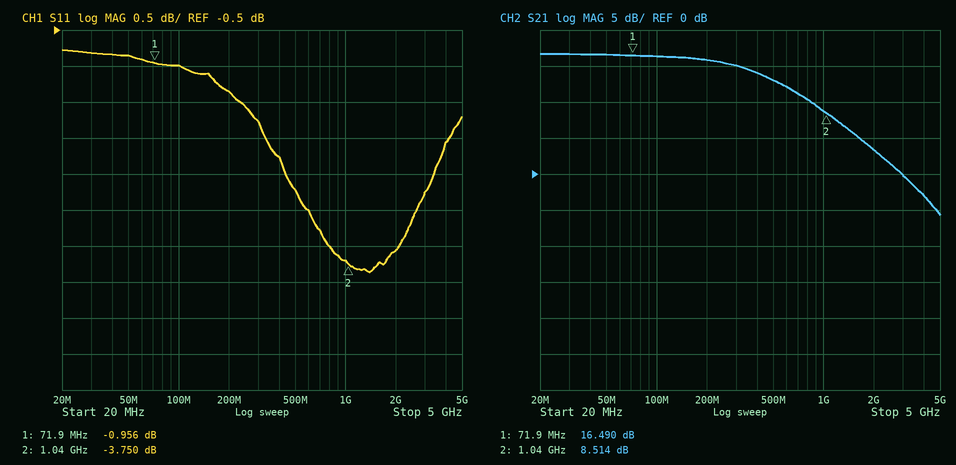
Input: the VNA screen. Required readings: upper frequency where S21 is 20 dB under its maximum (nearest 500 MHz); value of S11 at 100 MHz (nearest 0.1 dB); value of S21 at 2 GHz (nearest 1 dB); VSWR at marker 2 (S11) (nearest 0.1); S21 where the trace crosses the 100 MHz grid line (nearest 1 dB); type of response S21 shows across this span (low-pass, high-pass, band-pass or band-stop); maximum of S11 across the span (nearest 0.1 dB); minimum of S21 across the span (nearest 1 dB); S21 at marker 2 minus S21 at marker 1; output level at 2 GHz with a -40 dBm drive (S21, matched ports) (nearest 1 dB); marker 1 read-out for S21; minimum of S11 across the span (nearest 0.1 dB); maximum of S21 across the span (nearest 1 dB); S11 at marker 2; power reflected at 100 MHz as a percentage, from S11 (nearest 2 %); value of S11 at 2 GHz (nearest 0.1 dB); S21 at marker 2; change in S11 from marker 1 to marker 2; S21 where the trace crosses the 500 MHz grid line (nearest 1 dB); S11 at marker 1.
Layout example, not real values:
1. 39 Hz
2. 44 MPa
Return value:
1. 4.0 GHz
2. -1.0 dB
3. 3 dB
4. 4.7
5. 16 dB
6. low-pass
7. -0.8 dB
8. -6 dB
9. -7.976 dB
10. -37 dBm
11. 16.490 dB
12. -3.9 dB
13. 17 dB
14. -3.750 dB
15. 80 %
16. -3.6 dB
17. 8.514 dB
18. -2.794 dB
19. 13 dB
20. -0.956 dB
